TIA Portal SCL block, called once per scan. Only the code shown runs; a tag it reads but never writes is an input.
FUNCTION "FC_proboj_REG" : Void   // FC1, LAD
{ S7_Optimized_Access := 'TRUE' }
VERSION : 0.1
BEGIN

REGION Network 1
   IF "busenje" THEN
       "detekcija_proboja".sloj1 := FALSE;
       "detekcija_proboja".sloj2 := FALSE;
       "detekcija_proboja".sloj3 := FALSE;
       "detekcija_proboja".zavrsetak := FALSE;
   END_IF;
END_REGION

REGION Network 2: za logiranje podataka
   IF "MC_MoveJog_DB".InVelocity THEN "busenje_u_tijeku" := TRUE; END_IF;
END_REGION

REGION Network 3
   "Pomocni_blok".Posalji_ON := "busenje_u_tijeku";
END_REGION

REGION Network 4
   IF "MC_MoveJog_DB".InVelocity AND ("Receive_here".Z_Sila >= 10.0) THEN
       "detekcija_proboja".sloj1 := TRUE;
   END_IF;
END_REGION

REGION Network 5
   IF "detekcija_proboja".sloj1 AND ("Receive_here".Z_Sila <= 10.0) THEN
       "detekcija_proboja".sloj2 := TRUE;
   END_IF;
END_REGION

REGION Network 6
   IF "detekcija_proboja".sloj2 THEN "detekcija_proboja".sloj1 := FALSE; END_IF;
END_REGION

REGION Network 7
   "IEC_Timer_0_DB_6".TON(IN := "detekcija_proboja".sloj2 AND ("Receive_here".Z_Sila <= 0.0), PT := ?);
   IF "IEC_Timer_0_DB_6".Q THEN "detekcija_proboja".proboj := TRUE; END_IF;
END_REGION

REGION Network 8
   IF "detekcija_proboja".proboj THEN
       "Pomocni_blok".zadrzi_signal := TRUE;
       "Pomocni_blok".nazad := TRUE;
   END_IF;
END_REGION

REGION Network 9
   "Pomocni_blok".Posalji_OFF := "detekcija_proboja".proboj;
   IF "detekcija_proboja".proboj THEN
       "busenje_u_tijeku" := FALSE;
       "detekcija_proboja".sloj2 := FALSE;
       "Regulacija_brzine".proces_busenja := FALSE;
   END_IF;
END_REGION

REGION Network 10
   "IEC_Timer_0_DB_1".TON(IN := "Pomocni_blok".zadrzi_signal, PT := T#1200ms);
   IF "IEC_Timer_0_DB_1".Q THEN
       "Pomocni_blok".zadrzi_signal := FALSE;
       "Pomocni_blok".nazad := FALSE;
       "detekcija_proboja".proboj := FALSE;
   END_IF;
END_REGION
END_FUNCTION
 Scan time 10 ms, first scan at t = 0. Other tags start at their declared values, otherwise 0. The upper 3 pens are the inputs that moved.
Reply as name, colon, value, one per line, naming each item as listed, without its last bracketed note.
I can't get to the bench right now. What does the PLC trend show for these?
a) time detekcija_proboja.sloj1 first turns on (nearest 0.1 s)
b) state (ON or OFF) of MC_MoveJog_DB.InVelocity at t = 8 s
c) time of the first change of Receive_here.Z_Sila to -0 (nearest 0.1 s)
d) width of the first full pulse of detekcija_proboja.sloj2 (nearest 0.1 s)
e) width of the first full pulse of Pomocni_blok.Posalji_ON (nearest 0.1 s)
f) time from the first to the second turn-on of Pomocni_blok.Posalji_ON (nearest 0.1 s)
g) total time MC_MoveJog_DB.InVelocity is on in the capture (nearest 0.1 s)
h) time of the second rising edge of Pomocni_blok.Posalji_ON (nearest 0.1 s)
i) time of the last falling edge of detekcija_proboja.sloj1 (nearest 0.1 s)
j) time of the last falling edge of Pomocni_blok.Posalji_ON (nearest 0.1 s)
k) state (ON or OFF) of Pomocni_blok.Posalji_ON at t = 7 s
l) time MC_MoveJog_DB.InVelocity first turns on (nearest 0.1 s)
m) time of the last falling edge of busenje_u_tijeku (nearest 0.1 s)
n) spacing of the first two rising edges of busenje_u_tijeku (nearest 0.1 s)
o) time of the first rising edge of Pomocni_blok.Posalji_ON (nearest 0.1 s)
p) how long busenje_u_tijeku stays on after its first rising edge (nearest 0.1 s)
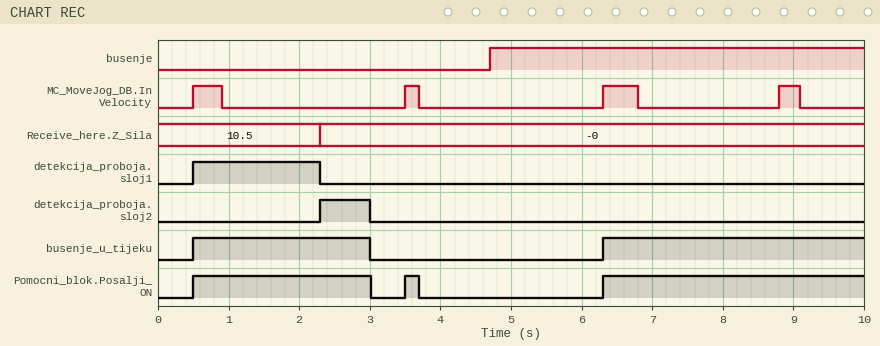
time detekcija_proboja.sloj1 first turns on: 0.5 s
state (ON or OFF) of MC_MoveJog_DB.InVelocity at t = 8 s: OFF
time of the first change of Receive_here.Z_Sila to -0: 2.3 s
width of the first full pulse of detekcija_proboja.sloj2: 0.7 s
width of the first full pulse of Pomocni_blok.Posalji_ON: 2.5 s
time from the first to the second turn-on of Pomocni_blok.Posalji_ON: 3.0 s
total time MC_MoveJog_DB.InVelocity is on in the capture: 1.4 s
time of the second rising edge of Pomocni_blok.Posalji_ON: 3.5 s
time of the last falling edge of detekcija_proboja.sloj1: 2.3 s
time of the last falling edge of Pomocni_blok.Posalji_ON: 3.7 s
state (ON or OFF) of Pomocni_blok.Posalji_ON at t = 7 s: ON
time MC_MoveJog_DB.InVelocity first turns on: 0.5 s
time of the last falling edge of busenje_u_tijeku: 3.0 s
spacing of the first two rising edges of busenje_u_tijeku: 5.8 s
time of the first rising edge of Pomocni_blok.Posalji_ON: 0.5 s
how long busenje_u_tijeku stays on after its first rising edge: 2.5 s
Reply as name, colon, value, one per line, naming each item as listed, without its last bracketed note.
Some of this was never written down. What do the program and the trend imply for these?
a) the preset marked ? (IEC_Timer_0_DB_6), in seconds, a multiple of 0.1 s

the preset marked ? (IEC_Timer_0_DB_6), in seconds, a multiple of 0.1 s: 0.7 s
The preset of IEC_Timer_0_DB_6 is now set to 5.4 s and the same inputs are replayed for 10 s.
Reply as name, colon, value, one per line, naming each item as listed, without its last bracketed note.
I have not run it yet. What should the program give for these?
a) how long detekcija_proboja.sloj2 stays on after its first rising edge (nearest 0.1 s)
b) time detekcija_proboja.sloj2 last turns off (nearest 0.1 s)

how long detekcija_proboja.sloj2 stays on after its first rising edge: 2.4 s
time detekcija_proboja.sloj2 last turns off: 4.7 s
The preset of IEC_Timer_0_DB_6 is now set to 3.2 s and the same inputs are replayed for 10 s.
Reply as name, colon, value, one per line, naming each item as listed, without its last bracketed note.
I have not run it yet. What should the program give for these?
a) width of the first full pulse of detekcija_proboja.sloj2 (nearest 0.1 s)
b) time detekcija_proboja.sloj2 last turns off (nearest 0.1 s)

width of the first full pulse of detekcija_proboja.sloj2: 2.4 s
time detekcija_proboja.sloj2 last turns off: 4.7 s
